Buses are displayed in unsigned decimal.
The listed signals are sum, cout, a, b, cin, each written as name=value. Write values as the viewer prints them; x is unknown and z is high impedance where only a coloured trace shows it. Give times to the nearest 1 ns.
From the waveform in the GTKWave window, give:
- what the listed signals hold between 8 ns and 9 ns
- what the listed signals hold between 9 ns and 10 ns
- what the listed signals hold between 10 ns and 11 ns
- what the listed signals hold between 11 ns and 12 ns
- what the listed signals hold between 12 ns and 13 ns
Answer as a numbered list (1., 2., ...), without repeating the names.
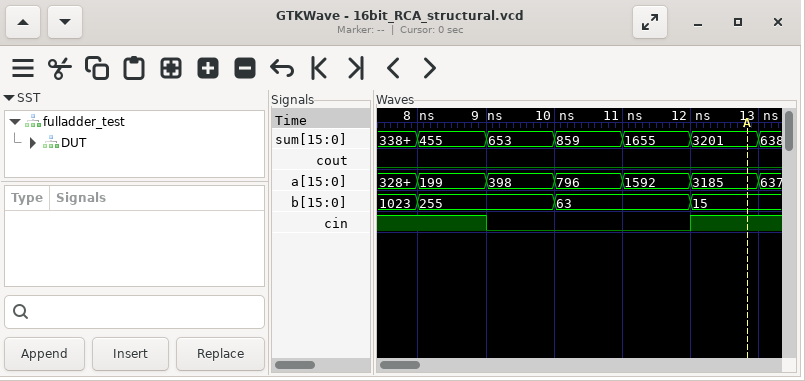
1. sum=455, cout=0, a=199, b=255, cin=1
2. sum=653, cout=0, a=398, b=255, cin=0
3. sum=859, cout=0, a=796, b=63, cin=0
4. sum=1655, cout=0, a=1592, b=63, cin=0
5. sum=3201, cout=0, a=3185, b=15, cin=1
